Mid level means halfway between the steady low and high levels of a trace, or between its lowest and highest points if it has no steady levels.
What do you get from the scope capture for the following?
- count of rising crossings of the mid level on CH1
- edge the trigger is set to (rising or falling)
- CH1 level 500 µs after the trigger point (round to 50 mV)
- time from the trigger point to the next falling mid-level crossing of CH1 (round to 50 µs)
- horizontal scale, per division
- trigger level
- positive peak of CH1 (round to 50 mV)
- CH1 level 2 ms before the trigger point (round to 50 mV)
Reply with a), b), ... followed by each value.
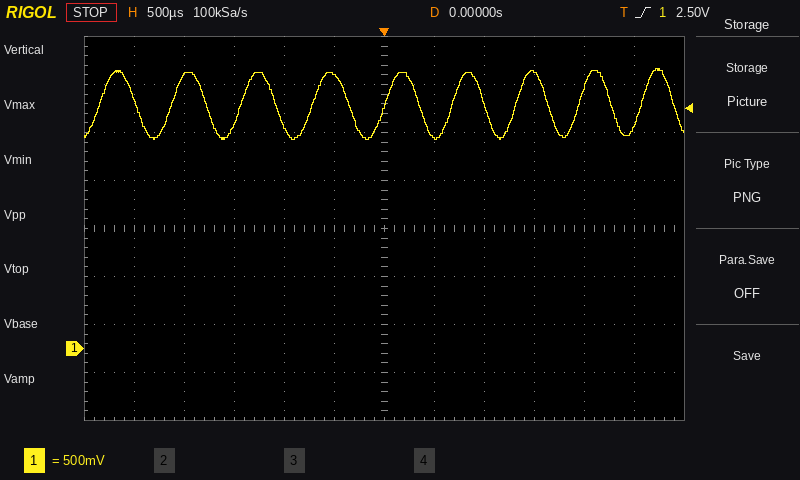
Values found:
a) 9
b) rising
c) 2.20 V
d) 350 µs
e) 500 µs
f) 2.50 V
g) 2.90 V
h) 2.85 V
